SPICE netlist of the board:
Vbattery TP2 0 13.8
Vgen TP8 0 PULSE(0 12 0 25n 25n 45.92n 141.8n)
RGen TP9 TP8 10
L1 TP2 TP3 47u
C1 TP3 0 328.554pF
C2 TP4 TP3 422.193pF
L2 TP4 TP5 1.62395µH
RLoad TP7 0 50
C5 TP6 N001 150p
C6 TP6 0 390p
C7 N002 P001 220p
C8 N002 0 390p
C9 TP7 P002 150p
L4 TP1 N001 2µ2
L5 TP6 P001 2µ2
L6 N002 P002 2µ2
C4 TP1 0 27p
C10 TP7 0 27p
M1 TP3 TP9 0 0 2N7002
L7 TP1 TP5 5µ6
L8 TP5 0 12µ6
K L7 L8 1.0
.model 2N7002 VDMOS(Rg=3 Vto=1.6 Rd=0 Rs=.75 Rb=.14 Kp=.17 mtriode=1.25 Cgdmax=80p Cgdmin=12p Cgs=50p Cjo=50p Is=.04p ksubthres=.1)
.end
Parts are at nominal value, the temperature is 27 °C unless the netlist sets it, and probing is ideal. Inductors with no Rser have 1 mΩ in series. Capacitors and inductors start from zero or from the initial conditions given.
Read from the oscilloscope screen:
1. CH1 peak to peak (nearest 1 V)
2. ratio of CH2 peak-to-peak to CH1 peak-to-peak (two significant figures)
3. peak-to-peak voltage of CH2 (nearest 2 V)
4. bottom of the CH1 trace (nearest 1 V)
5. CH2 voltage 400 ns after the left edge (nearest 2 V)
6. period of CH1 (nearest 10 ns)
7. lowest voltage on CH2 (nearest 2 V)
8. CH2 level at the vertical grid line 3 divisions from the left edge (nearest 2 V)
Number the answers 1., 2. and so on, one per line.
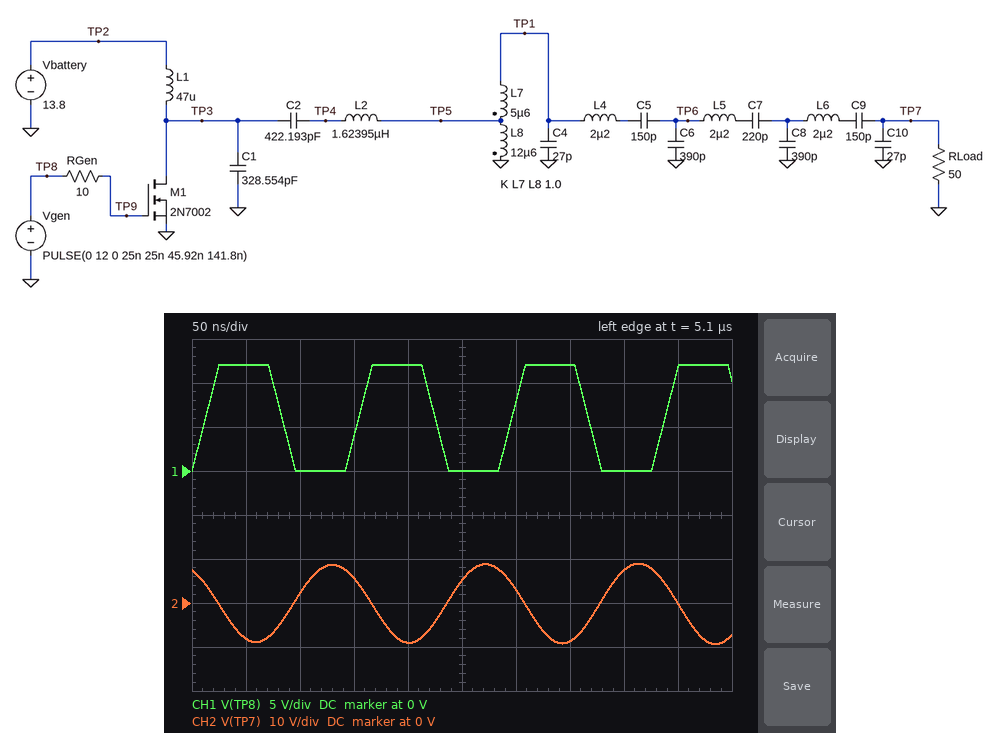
1. 12 V
2. 1.5
3. 18 V
4. 0 V
5. 8 V
6. 140 ns
7. -10 V
8. 6 V
